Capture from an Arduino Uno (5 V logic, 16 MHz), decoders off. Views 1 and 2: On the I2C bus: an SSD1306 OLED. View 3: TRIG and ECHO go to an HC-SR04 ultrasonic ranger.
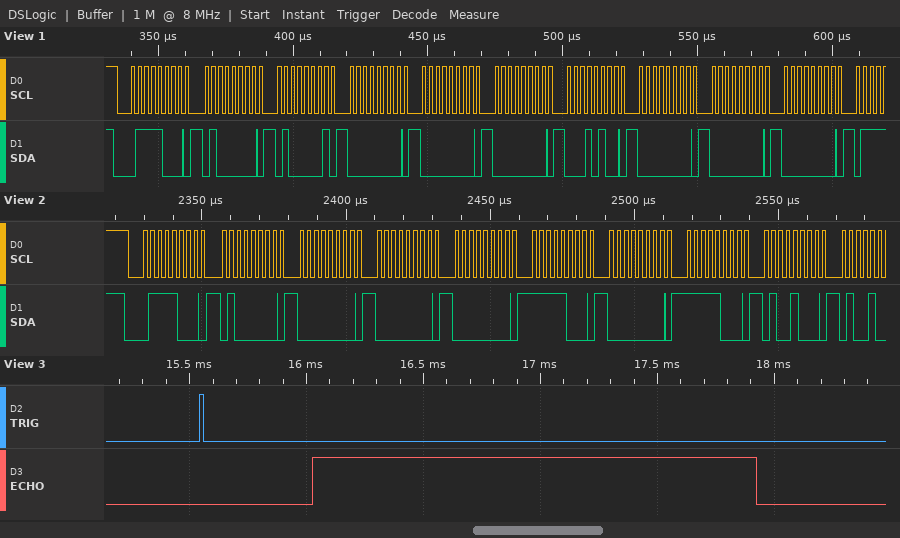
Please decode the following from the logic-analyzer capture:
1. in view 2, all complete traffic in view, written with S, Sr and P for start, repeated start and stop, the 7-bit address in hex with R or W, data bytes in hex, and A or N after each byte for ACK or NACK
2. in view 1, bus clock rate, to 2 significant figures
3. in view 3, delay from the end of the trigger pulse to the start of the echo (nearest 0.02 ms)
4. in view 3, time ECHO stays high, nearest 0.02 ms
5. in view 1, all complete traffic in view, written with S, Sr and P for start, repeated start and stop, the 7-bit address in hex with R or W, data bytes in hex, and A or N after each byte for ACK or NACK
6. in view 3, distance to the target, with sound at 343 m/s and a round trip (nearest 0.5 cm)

S 3CW A 40 A 00 A 00 A 00 A F8 A 00 A F8 A 48 A
400 kHz
0.46 ms
1.90 ms
S 3CW A 40 A 41 A 00 A 00 A 00 A 14 A 00 A 00 A 00 A
32.5 cm
